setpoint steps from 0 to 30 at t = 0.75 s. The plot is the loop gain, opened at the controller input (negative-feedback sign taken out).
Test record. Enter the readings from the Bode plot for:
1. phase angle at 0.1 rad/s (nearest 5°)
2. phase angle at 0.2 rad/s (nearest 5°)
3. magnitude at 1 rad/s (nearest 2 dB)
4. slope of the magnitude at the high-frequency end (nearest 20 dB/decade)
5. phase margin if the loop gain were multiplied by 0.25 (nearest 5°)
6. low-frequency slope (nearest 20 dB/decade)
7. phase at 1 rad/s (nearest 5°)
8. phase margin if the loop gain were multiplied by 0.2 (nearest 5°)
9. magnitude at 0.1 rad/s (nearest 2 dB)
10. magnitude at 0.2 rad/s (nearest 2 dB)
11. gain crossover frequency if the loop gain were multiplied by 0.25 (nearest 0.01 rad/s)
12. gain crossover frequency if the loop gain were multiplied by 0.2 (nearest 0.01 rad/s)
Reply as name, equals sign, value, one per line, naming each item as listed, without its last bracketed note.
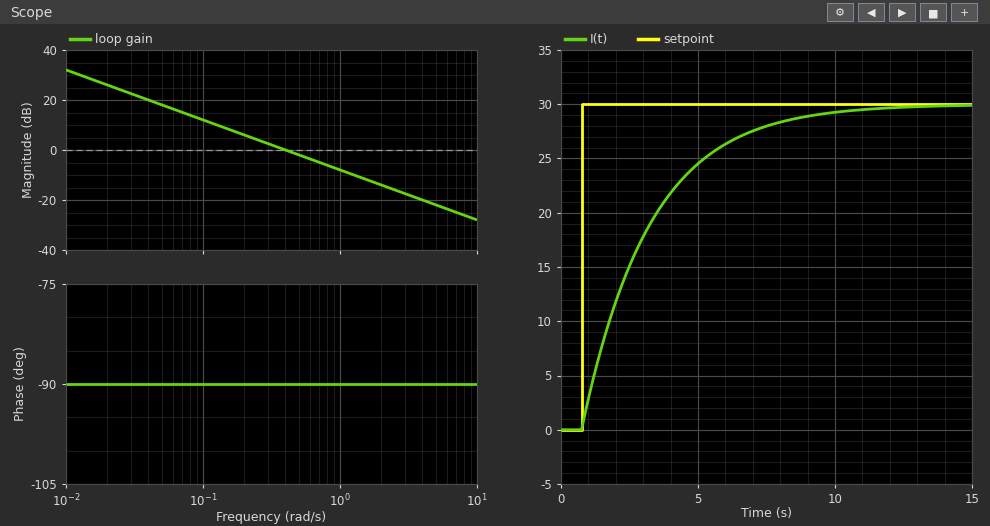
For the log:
phase angle at 0.1 rad/s = -90°
phase angle at 0.2 rad/s = -90°
magnitude at 1 rad/s = -8 dB
slope of the magnitude at the high-frequency end = -20 dB/decade
phase margin if the loop gain were multiplied by 0.25 = 90°
low-frequency slope = -20 dB/decade
phase at 1 rad/s = -90°
phase margin if the loop gain were multiplied by 0.2 = 90°
magnitude at 0.1 rad/s = 12 dB
magnitude at 0.2 rad/s = 6 dB
gain crossover frequency if the loop gain were multiplied by 0.25 = 0.10 rad/s
gain crossover frequency if the loop gain were multiplied by 0.2 = 0.08 rad/s
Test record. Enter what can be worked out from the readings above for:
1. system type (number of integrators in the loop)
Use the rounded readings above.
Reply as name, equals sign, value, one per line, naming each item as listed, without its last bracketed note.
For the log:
system type = 1
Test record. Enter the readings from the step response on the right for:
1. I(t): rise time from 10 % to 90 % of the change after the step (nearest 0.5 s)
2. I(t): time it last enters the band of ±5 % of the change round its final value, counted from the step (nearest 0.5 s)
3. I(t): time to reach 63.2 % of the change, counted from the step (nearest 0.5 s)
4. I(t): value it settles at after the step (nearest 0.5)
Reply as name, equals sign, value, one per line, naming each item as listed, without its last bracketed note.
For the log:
I(t): rise time from 10 % to 90 % of the change after the step = 5.5 s
I(t): time it last enters the band of ±5 % of the change round its final value, counted from the step = 7.5 s
I(t): time to reach 63.2 % of the change, counted from the step = 2.5 s
I(t): value it settles at after the step = 30.0
